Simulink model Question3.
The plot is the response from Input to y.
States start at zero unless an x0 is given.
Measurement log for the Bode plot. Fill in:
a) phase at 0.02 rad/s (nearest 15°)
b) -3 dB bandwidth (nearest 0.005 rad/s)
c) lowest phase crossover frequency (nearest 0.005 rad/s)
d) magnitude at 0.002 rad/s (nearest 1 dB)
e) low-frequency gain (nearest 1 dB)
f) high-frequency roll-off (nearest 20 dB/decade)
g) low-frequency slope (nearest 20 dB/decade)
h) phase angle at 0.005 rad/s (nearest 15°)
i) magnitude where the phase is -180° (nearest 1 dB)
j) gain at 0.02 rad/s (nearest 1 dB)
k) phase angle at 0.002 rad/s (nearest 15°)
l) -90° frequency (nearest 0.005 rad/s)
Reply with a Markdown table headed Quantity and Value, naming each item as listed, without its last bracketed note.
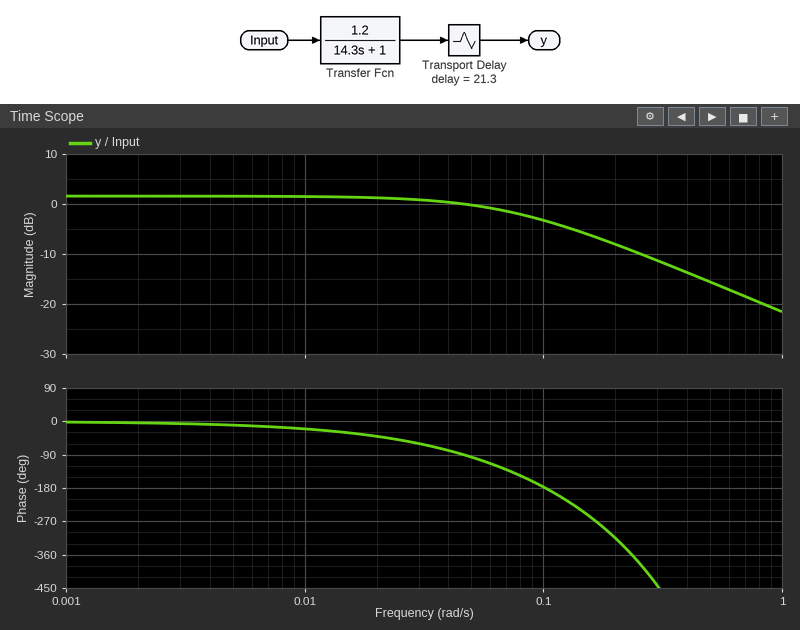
| Quantity | Value |
|---|---|
| phase at 0.02 rad/s | -45° |
| -3 dB bandwidth | 0.070 rad/s |
| lowest phase crossover frequency | 0.100 rad/s |
| magnitude at 0.002 rad/s | 2 dB |
| low-frequency gain | 2 dB |
| high-frequency roll-off | -20 dB/decade |
| low-frequency slope | 0 dB/decade |
| phase angle at 0.005 rad/s | -15° |
| magnitude where the phase is -180° | -3 dB |
| gain at 0.02 rad/s | 1 dB |
| phase angle at 0.002 rad/s | 0° |
| -90° frequency | 0.045 rad/s |
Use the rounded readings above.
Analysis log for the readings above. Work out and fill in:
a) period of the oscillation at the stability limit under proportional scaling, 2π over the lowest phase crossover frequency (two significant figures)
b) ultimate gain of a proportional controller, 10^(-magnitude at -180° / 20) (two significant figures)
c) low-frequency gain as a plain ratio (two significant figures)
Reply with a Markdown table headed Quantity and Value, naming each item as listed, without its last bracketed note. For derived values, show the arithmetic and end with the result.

| Quantity | Value |
|---|---|
| period of the oscillation at the stability limit under proportional scaling, 2π over the lowest phase crossover frequency | 2π / 0.1 = 63 s |
| ultimate gain of a proportional controller, 10^(-magnitude at -180° / 20) | 10^(3 / 20) = 1.4 |
| low-frequency gain as a plain ratio | 10^(2 / 20) = 1.3 |
